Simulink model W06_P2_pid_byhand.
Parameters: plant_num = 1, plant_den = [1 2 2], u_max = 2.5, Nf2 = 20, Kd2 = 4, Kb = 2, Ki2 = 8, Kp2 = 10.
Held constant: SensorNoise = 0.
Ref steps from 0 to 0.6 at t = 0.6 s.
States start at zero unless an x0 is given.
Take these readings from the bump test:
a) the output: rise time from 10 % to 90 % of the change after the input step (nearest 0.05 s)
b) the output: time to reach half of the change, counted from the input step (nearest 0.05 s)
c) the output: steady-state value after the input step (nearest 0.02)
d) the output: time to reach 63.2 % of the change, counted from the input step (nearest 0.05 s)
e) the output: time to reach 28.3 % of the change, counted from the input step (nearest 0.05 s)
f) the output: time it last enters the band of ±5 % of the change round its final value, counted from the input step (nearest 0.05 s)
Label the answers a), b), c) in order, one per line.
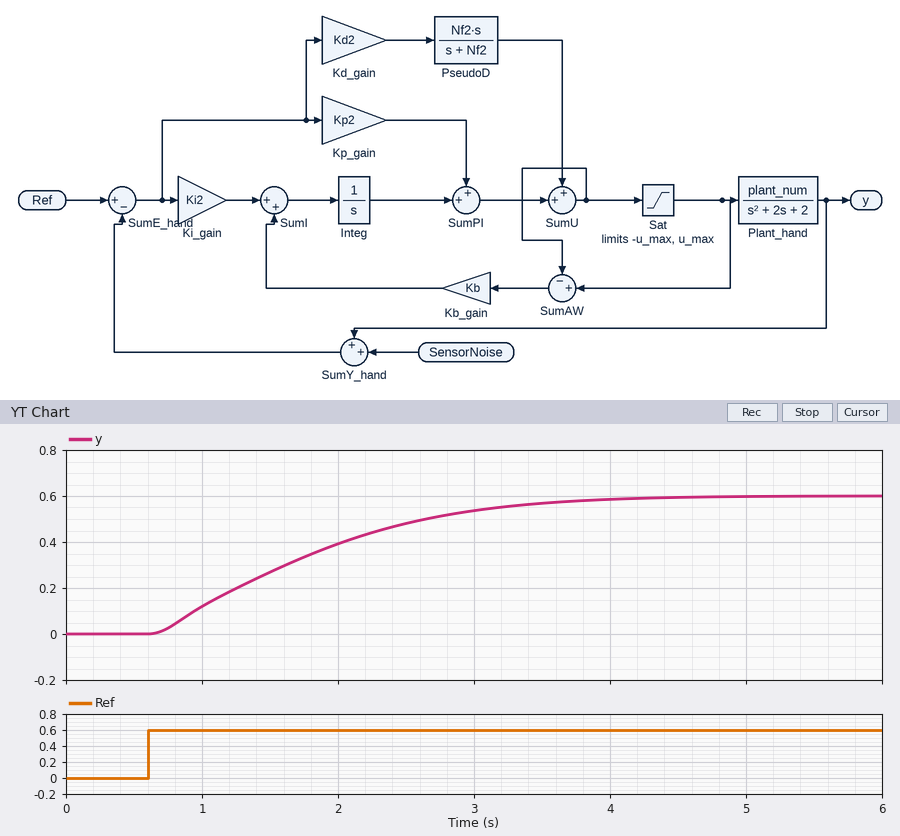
a) 2.20 s
b) 1.00 s
c) 0.60
d) 1.35 s
e) 0.55 s
f) 2.95 s
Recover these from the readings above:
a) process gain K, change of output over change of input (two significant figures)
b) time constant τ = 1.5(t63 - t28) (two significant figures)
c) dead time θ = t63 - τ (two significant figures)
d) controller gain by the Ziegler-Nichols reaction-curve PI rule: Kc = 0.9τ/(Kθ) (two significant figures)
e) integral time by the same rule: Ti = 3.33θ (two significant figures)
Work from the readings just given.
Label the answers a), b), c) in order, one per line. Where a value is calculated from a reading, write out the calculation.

a) (0.6 - 0) / 0.6 = 1.0
b) 1.5 × (1.35 - 0.55) = 1.2 s
c) 1.35 - 1.2 = 0.15 s
d) 0.9 × 1.2 / (1 × 0.15) = 7.2
e) 3.33 × 0.15 = 0.50 s
